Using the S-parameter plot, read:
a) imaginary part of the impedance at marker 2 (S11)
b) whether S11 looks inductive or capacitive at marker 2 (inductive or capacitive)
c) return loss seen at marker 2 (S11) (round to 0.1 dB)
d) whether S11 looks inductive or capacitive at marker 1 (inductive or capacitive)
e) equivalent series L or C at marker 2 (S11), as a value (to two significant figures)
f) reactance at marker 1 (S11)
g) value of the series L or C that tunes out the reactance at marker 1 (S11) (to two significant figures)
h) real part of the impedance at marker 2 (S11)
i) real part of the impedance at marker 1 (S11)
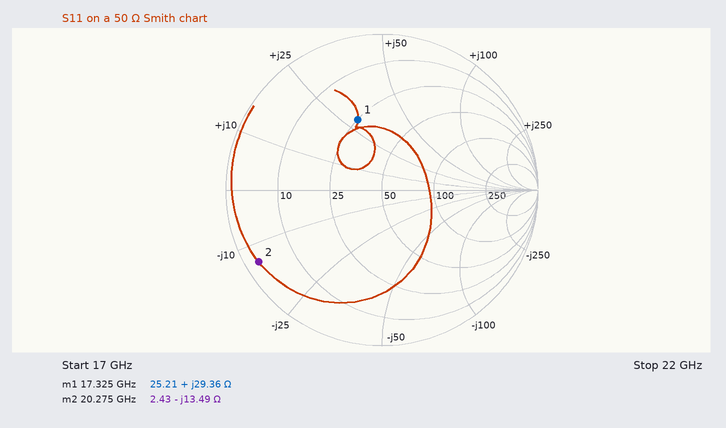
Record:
-13.49 Ω
capacitive
0.8 dB
inductive
580 fF
+29.36 Ω
310 fF
2.43 Ω
25.21 Ω
